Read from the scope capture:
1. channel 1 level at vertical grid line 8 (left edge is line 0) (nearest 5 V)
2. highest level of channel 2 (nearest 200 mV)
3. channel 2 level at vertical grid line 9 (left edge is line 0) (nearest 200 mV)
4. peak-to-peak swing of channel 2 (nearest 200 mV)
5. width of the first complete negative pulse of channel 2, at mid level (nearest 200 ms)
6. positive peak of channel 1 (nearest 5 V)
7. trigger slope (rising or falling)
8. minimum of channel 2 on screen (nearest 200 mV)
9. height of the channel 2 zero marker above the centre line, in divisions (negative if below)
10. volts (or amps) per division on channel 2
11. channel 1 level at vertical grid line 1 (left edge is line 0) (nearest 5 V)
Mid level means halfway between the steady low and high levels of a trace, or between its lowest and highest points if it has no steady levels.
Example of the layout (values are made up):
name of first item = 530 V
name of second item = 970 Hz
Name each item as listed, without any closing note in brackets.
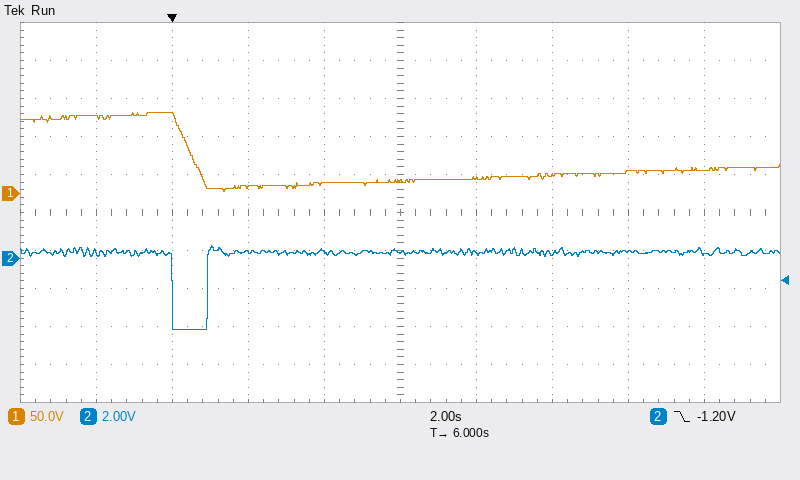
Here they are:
channel 1 level at vertical grid line 8 (left edge is line 0) = 30 V
highest level of channel 2 = 600 mV
channel 2 level at vertical grid line 9 (left edge is line 0) = 400 mV
peak-to-peak swing of channel 2 = 4.4 V
width of the first complete negative pulse of channel 2, at mid level = 1.0 s
positive peak of channel 1 = 105 V
trigger slope = falling
minimum of channel 2 on screen = -3.8 V
height of the channel 2 zero marker above the centre line, in divisions = -1.2 div
volts (or amps) per division on channel 2 = 2 V
channel 1 level at vertical grid line 1 (left edge is line 0) = 100 V
